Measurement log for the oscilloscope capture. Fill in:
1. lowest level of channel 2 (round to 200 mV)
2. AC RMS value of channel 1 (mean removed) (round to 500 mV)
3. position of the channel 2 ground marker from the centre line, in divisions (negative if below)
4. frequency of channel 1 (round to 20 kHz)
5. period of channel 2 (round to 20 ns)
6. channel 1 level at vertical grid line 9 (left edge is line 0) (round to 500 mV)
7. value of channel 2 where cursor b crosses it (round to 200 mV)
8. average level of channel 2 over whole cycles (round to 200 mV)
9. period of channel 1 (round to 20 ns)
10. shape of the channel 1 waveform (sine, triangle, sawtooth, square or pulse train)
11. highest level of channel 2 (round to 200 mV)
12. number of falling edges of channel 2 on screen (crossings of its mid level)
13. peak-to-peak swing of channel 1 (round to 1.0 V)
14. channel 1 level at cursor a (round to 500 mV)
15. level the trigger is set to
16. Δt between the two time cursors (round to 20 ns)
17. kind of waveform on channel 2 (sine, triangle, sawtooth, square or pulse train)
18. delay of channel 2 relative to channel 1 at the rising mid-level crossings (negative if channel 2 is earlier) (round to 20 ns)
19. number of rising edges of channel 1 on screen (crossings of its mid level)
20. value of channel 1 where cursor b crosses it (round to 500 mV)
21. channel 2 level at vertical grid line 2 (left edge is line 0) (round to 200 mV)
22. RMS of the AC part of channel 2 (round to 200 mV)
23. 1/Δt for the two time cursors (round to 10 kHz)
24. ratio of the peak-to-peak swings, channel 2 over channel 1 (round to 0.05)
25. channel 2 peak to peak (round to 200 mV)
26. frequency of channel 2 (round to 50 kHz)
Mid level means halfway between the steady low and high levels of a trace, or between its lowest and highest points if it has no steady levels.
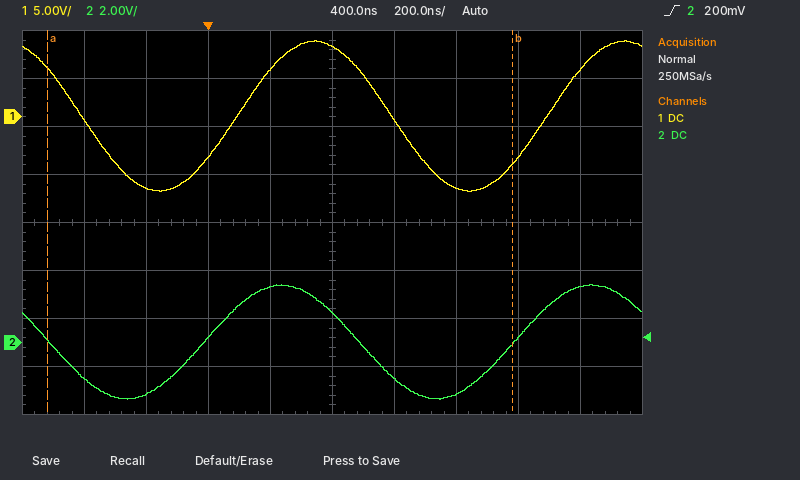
-2.4 V
5.5 V
-2.5 div
1.00 MHz
1.00 µs
5.0 V
0.0 V
0.0 V
1.00 µs
sine
2.4 V
2
16.0 V
5.0 V
200 mV
1.50 µs
sine
-100 ns
2
-5.0 V
-2.2 V
1.6 V
670 kHz
0.30
4.8 V
1.00 MHz
